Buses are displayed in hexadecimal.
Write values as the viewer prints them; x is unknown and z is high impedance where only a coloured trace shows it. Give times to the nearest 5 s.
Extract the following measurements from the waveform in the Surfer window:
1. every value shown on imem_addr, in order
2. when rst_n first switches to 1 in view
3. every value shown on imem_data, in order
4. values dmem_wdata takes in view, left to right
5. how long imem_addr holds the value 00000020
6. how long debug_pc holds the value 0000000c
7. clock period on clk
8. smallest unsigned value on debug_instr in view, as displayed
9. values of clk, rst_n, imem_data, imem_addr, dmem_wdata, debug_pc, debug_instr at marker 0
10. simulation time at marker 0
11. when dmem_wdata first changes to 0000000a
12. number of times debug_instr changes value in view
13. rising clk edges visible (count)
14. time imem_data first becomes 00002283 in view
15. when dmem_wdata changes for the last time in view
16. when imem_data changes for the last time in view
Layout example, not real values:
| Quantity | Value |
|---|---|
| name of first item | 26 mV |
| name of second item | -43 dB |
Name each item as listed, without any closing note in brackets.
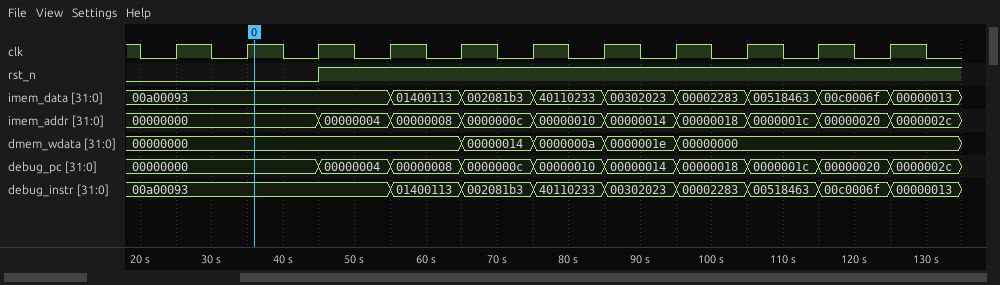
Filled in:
| Quantity | Value |
|---|---|
| every value shown on imem_addr, in order | 00000000, 00000004, 00000008, 0000000c, 00000010, 00000014, 00000018, 0000001c, 00000020, 0000002c |
| when rst_n first switches to 1 in view | 45 s |
| every value shown on imem_data, in order | 00a00093, 01400113, 002081b3, 40110233, 00302023, 00002283, 00518463, 00c0006f, 00000013 |
| values dmem_wdata takes in view, left to right | 00000000, 00000014, 0000000a, 0000001e, 00000000 |
| how long imem_addr holds the value 00000020 | 10 s |
| how long debug_pc holds the value 0000000c | 10 s |
| clock period on clk | 10 s |
| smallest unsigned value on debug_instr in view, as displayed | 00000013 |
| values of clk, rst_n, imem_data, imem_addr, dmem_wdata, debug_pc, debug_instr at marker 0 | clk=1, rst_n=0, imem_data=00a00093, imem_addr=00000000, dmem_wdata=00000000, debug_pc=00000000, debug_instr=00a00093 |
| simulation time at marker 0 | 35 s |
| when dmem_wdata first changes to 0000000a | 75 s |
| number of times debug_instr changes value in view | 8 |
| rising clk edges visible | 11 |
| time imem_data first becomes 00002283 in view | 95 s |
| when dmem_wdata changes for the last time in view | 95 s |
| when imem_data changes for the last time in view | 125 s |
